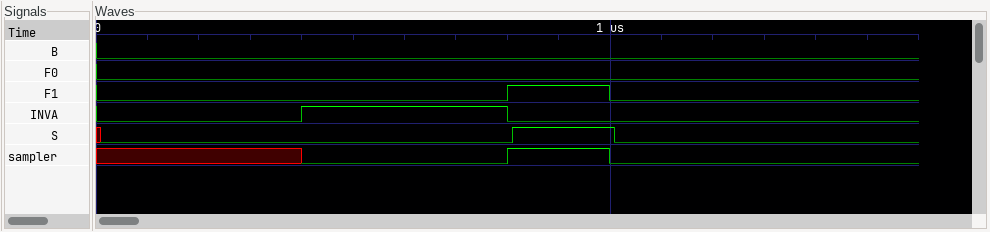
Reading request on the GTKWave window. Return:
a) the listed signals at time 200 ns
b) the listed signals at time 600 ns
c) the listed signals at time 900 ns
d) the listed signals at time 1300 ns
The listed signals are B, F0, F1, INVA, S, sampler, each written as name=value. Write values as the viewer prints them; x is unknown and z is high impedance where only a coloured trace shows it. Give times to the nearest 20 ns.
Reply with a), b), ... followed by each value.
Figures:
a) B=0, F0=0, F1=0, INVA=0, S=0, sampler=x
b) B=0, F0=0, F1=0, INVA=1, S=0, sampler=0
c) B=0, F0=0, F1=1, INVA=0, S=1, sampler=1
d) B=0, F0=0, F1=0, INVA=0, S=0, sampler=0
